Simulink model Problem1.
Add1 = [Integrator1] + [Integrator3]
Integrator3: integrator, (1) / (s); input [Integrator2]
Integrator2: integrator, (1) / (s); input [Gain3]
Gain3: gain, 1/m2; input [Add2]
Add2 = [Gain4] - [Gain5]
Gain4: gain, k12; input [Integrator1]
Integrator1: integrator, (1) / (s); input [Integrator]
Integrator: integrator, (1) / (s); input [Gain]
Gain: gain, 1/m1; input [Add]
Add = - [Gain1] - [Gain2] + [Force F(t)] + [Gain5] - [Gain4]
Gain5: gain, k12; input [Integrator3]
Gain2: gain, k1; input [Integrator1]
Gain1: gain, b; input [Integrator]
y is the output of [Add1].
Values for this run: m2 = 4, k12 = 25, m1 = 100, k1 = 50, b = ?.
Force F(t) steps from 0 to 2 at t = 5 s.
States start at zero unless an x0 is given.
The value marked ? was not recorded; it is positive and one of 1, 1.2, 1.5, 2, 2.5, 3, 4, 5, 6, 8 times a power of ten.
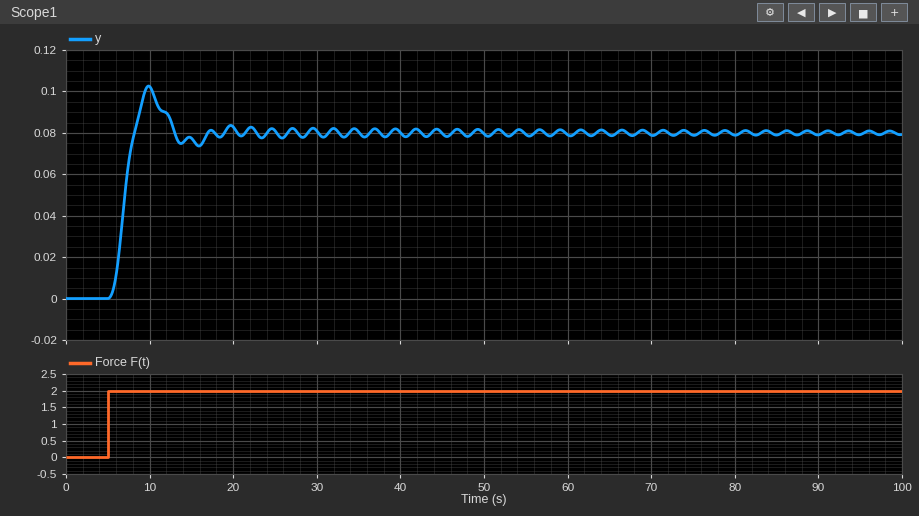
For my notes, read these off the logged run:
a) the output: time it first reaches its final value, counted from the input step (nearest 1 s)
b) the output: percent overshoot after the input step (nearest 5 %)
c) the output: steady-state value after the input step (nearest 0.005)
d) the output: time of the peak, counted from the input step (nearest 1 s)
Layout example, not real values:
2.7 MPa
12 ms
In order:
3 s
30 %
0.080
5 s
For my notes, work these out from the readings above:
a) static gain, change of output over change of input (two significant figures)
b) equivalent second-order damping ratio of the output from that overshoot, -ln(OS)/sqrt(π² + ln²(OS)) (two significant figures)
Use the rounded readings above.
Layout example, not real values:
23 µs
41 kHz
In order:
0.040
0.36
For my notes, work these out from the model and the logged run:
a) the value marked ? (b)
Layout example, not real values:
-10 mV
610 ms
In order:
60
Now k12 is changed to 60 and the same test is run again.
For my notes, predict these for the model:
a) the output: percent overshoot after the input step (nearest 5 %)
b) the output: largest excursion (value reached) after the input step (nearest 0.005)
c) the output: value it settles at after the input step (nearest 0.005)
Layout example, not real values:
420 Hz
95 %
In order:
25 %
0.100
0.080
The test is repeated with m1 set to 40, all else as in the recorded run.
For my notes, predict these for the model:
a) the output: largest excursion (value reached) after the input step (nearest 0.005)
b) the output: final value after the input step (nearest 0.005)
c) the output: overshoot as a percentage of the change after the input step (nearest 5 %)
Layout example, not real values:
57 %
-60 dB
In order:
0.090
0.080
10 %
